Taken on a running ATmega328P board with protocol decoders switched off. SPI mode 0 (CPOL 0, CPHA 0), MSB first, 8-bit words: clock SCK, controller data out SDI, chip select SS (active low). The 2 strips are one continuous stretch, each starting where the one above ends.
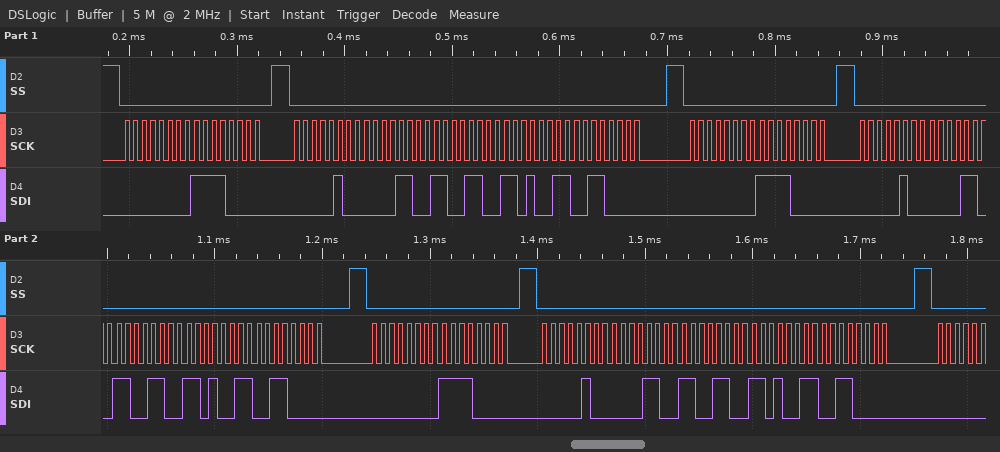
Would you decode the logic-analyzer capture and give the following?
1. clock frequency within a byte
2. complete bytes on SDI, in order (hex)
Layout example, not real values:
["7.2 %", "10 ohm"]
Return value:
["125 kHz", "00 F0 04 0C CC D3 30 00 F0 04 0C CC D3 30 00 F0 04 0C CC D3 30"]
